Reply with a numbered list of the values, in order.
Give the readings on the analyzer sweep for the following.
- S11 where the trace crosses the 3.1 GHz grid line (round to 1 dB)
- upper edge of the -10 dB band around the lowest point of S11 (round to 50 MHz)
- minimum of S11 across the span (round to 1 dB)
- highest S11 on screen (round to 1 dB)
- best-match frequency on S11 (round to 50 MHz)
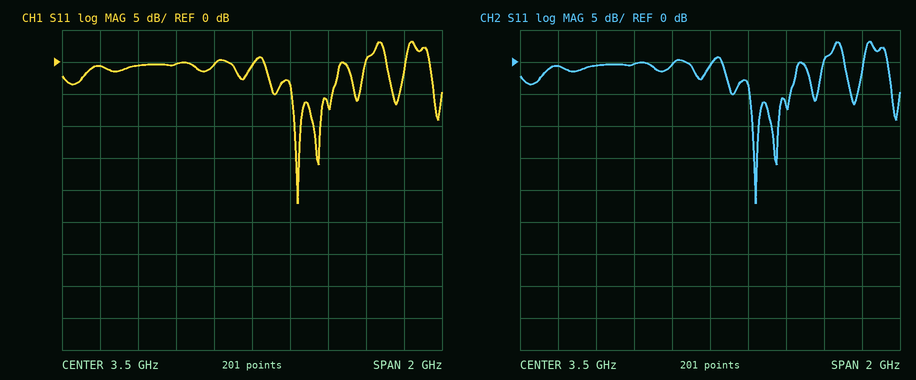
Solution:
1. 0 dB
2. 3.75 GHz
3. -22 dB
4. 3 dB
5. 3.75 GHz
